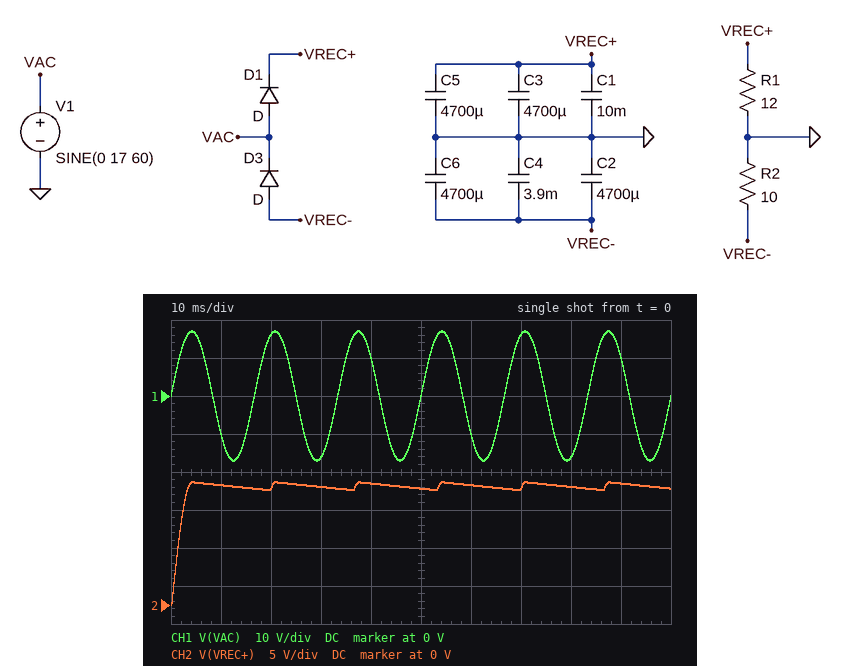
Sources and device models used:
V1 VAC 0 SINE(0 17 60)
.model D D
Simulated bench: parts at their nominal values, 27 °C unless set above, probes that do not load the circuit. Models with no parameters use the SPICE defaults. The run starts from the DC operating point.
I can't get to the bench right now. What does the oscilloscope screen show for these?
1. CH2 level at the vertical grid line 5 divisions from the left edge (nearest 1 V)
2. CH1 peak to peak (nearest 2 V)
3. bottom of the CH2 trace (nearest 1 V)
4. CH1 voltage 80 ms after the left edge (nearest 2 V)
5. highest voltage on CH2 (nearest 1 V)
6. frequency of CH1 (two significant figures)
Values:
15 V
34 V
0 V
-16 V
16 V
60 Hz
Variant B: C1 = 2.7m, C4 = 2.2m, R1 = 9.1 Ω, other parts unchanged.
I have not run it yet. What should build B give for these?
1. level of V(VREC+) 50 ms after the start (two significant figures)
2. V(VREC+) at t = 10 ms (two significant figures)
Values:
14 V
15 V
